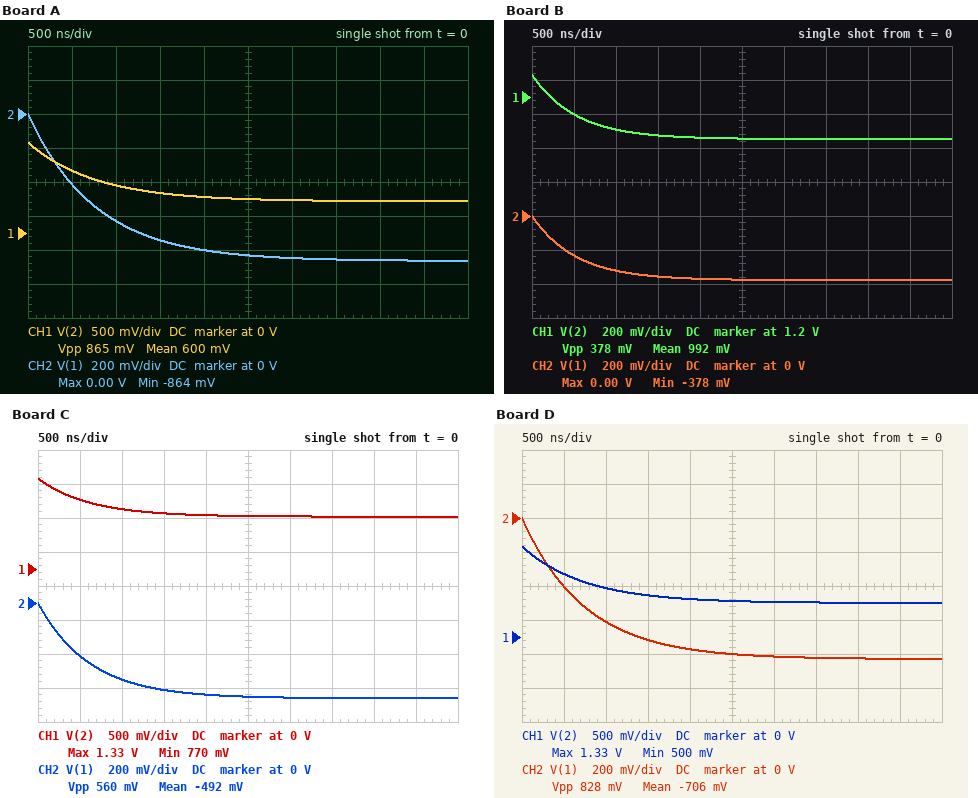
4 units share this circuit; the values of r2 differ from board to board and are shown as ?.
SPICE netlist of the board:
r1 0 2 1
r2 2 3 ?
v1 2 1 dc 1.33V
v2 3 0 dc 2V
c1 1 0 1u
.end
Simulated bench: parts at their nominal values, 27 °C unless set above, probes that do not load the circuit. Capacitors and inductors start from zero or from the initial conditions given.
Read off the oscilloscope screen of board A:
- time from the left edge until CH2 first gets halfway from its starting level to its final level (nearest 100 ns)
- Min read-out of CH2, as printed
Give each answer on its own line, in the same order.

500 ns
-864 mV
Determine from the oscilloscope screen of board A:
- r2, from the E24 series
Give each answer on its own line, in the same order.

3.3 Ω
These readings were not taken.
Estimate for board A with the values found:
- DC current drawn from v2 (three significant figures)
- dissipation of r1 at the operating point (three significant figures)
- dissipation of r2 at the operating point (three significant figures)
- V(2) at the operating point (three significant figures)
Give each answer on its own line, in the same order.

465 mA
216 mW
714 mW
465 mV
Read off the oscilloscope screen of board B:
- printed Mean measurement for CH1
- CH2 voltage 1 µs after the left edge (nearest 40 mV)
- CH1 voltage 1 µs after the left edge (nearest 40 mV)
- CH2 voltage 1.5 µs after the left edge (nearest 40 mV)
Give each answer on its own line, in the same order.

992 mV
-320 mV
1.00 V
-360 mV
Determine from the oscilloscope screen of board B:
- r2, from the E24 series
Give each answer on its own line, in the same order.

1.1 Ω
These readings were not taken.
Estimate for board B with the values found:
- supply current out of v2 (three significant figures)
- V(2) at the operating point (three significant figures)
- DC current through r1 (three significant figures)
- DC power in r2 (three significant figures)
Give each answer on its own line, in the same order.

952 mA
952 mV
952 mA
998 mW
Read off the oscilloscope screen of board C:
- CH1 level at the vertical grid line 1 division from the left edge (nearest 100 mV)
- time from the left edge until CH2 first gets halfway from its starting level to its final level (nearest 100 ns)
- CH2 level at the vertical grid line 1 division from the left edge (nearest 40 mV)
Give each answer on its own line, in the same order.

1.0 V
400 ns
-320 mV
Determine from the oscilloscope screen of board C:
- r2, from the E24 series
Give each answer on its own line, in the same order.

1.6 Ω
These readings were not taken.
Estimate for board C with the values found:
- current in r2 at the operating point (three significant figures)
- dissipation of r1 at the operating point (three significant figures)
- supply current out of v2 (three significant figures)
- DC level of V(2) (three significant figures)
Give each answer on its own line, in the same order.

769 mA
592 mW
769 mA
769 mV
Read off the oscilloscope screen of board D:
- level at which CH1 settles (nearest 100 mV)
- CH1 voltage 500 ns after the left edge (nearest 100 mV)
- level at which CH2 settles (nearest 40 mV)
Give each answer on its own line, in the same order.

500 mV
900 mV
-840 mV
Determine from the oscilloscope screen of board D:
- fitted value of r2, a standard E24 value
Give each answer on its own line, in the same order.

3 Ω
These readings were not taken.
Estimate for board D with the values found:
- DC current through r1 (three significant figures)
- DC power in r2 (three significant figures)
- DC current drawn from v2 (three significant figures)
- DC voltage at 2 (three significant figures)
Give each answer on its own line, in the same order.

500 mA
750 mW
500 mA
500 mV
